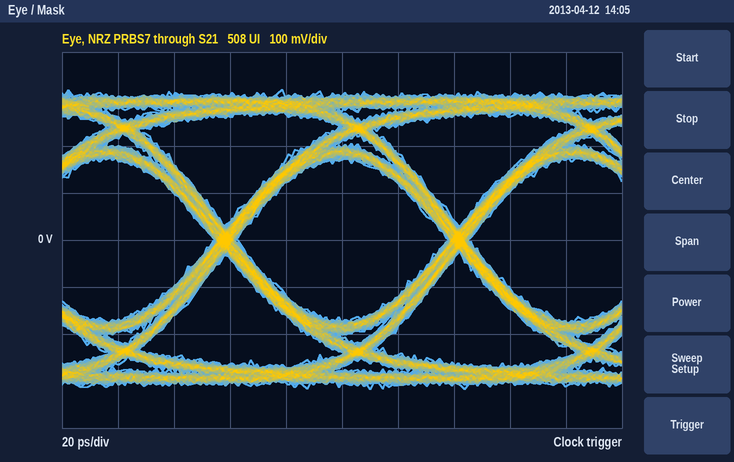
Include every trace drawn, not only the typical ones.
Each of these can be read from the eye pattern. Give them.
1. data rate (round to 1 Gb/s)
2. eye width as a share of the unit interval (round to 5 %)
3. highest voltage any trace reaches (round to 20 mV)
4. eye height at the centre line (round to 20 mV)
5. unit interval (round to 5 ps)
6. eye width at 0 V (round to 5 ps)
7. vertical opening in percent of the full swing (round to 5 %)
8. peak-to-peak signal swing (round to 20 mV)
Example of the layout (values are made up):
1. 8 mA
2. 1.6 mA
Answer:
1. 12 Gb/s
2. 90 %
3. 320 mV
4. 340 mV
5. 85 ps
6. 75 ps
7. 55 %
8. 640 mV
